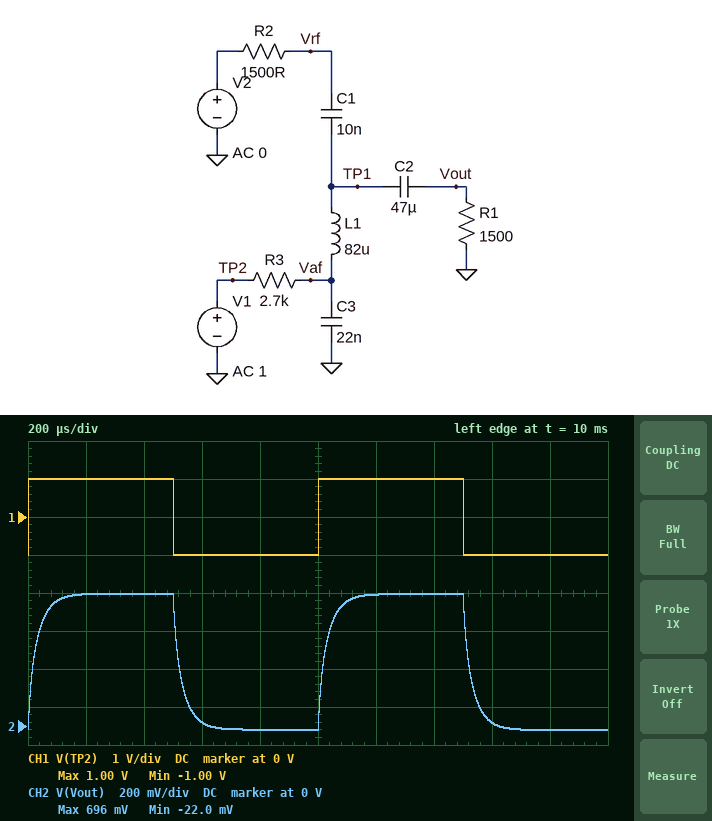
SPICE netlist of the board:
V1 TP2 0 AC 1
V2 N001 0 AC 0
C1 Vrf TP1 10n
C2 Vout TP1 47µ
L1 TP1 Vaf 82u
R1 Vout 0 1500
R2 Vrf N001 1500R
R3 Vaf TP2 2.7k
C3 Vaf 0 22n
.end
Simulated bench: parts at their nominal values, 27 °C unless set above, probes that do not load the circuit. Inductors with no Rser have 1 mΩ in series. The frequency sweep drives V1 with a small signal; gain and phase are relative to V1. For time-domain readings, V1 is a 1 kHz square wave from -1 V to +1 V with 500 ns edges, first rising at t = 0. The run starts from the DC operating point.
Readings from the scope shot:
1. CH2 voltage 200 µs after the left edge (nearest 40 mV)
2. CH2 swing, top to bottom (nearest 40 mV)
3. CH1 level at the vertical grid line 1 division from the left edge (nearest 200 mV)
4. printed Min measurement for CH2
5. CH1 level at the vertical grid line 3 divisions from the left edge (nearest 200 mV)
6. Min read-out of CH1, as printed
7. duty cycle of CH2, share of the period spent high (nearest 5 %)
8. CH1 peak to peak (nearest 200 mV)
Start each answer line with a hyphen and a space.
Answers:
- 680 mV
- 720 mV
- 1.0 V
- -22.0 mV
- -1.0 V
- -1.00 V
- 50 %
- 2.0 V
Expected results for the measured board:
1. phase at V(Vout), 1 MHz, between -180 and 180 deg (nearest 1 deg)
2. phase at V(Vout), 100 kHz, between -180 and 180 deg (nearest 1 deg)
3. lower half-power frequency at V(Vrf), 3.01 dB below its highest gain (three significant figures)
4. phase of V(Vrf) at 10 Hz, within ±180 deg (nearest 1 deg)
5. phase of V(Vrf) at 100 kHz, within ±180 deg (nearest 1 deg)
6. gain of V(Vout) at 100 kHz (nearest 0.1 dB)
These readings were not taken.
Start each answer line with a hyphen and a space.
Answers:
- -124 deg
- -87 deg
- 3.07 kHz
- 82 deg
- -81 deg
- -31.5 dB
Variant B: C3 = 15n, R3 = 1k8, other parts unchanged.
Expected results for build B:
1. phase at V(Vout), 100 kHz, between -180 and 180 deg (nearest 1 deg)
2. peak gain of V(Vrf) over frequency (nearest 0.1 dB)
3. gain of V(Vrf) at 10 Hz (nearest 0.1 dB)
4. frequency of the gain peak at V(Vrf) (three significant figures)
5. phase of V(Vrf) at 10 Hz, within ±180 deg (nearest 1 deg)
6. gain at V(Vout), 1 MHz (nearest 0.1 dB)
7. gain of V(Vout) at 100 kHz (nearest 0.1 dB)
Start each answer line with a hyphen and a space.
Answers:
- -83 deg
- -14.3 dB
- -67.2 dB
- 11.8 kHz
- 83 deg
- -46.2 dB
- -24.7 dB
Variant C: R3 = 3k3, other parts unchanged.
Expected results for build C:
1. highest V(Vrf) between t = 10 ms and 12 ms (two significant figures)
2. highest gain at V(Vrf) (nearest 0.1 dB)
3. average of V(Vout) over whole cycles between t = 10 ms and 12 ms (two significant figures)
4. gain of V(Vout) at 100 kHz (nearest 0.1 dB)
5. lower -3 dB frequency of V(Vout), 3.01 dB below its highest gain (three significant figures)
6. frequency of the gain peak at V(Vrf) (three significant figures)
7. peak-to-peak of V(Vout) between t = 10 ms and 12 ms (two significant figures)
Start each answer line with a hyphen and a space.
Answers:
- 160 mV
- -20.2 dB
- 300 mV
- -33.2 dB
- 705 mHz
- 8.67 kHz
- 630 mV
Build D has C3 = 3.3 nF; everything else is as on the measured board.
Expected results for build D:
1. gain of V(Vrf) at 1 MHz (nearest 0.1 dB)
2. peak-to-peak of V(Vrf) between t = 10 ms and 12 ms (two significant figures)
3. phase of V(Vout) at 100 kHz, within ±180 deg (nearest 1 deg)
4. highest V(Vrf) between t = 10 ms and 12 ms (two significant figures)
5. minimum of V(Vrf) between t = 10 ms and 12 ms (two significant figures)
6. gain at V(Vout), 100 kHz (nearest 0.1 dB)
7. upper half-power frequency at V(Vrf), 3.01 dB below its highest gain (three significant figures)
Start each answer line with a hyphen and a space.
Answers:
- -36.4 dB
- 680 mV
- -54 deg
- 340 mV
- -340 mV
- -17.1 dB
- 102 kHz
